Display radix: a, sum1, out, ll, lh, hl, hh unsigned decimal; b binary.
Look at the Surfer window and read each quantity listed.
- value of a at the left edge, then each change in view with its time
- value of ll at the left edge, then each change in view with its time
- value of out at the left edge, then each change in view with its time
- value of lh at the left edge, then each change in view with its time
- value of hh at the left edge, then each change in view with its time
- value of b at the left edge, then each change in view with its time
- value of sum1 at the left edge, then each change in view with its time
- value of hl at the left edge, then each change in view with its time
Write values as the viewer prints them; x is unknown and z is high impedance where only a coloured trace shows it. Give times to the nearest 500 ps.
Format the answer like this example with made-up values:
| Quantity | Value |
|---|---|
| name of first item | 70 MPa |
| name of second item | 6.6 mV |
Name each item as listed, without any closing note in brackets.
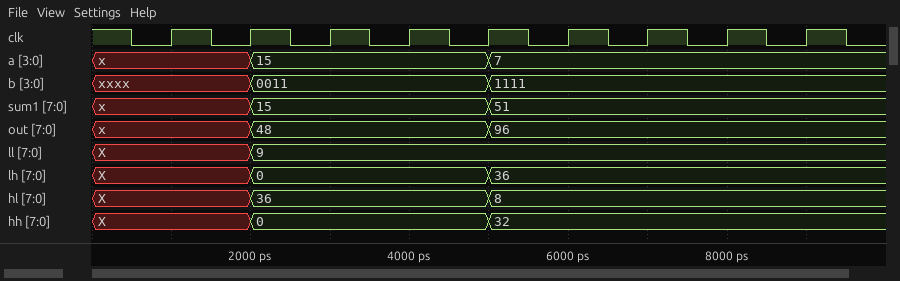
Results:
| Quantity | Value |
|---|---|
| value of a at the left edge, then each change in view with its time | x, 15 at 2000 ps, 7 at 5000 ps |
| value of ll at the left edge, then each change in view with its time | X, 9 at 2000 ps |
| value of out at the left edge, then each change in view with its time | x, 48 at 2000 ps, 96 at 5000 ps |
| value of lh at the left edge, then each change in view with its time | X, 0 at 2000 ps, 36 at 5000 ps |
| value of hh at the left edge, then each change in view with its time | X, 0 at 2000 ps, 32 at 5000 ps |
| value of b at the left edge, then each change in view with its time | xxxx, 0011 at 2000 ps, 1111 at 5000 ps |
| value of sum1 at the left edge, then each change in view with its time | x, 15 at 2000 ps, 51 at 5000 ps |
| value of hl at the left edge, then each change in view with its time | X, 36 at 2000 ps, 8 at 5000 ps |
